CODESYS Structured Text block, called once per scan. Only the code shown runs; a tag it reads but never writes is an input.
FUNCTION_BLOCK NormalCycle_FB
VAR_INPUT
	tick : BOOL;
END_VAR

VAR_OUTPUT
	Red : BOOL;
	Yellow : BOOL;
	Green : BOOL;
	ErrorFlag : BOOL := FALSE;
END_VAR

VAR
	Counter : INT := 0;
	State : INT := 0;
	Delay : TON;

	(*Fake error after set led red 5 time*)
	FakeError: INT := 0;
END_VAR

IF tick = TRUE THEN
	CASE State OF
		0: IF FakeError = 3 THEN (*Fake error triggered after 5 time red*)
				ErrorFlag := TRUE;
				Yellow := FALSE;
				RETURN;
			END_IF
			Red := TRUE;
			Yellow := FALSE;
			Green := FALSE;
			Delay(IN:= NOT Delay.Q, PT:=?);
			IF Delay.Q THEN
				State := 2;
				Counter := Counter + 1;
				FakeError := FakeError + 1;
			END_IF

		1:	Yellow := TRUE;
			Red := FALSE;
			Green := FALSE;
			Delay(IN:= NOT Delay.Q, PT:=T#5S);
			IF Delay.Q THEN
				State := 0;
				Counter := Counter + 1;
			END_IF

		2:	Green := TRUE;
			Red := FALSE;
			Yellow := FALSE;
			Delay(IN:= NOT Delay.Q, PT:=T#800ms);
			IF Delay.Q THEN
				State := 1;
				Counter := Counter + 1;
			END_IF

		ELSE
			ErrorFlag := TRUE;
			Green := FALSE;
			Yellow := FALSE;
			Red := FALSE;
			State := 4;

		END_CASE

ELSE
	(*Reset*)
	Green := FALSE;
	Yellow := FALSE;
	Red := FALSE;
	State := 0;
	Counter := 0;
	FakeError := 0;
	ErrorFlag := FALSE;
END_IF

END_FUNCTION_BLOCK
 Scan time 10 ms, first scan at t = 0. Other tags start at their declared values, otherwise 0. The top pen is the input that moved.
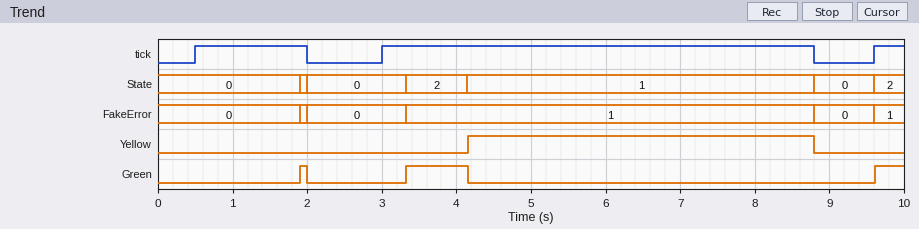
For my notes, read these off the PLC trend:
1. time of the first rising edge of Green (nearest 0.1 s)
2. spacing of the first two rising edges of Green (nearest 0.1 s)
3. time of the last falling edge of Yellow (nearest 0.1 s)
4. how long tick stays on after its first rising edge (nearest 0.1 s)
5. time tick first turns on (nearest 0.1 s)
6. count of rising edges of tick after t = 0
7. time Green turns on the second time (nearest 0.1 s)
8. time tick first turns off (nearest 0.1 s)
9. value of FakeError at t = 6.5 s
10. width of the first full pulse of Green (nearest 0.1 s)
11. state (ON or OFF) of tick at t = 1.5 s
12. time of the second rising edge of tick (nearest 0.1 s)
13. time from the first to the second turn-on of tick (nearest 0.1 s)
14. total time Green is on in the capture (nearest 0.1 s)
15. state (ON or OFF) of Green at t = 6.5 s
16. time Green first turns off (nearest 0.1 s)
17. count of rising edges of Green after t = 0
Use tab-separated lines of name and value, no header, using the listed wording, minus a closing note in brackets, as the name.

time of the first rising edge of Green	1.9 s
spacing of the first two rising edges of Green	1.4 s
time of the last falling edge of Yellow	8.8 s
how long tick stays on after its first rising edge	1.5 s
time tick first turns on	0.5 s
count of rising edges of tick after t = 0	3
time Green turns on the second time	3.3 s
time tick first turns off	2.0 s
value of FakeError at t = 6.5 s	1
width of the first full pulse of Green	0.1 s
state (ON or OFF) of tick at t = 1.5 s	ON
time of the second rising edge of tick	3.0 s
time from the first to the second turn-on of tick	2.5 s
total time Green is on in the capture	1.3 s
state (ON or OFF) of Green at t = 6.5 s	OFF
time Green first turns off	2.0 s
count of rising edges of Green after t = 0	3
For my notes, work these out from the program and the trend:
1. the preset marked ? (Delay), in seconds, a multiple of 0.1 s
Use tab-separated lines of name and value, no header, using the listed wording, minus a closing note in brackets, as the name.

the preset marked ? (Delay), in seconds, a multiple of 0.1 s	1.4 s
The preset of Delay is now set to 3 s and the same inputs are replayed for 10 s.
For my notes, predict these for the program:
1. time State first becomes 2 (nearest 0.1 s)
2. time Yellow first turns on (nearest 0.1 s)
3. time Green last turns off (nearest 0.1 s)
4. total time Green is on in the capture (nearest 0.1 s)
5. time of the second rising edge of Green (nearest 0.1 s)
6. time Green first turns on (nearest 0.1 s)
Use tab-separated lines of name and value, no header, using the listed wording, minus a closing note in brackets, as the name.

time State first becomes 2	3.5 s
time Yellow first turns on	4.3 s
time Green last turns off	4.3 s
total time Green is on in the capture	1.2 s
time of the second rising edge of Green	9.6 s
time Green first turns on	3.5 s
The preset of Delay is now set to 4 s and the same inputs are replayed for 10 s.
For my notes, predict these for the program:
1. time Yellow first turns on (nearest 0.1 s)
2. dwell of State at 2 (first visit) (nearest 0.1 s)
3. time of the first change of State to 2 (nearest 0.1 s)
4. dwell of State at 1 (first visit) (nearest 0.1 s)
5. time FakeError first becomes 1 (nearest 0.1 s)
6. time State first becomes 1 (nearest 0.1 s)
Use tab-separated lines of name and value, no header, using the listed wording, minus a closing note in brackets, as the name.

time Yellow first turns on	5.3 s
dwell of State at 2 (first visit)	0.8 s
time of the first change of State to 2	4.5 s
dwell of State at 1 (first visit)	3.5 s
time FakeError first becomes 1	4.5 s
time State first becomes 1	5.3 s
